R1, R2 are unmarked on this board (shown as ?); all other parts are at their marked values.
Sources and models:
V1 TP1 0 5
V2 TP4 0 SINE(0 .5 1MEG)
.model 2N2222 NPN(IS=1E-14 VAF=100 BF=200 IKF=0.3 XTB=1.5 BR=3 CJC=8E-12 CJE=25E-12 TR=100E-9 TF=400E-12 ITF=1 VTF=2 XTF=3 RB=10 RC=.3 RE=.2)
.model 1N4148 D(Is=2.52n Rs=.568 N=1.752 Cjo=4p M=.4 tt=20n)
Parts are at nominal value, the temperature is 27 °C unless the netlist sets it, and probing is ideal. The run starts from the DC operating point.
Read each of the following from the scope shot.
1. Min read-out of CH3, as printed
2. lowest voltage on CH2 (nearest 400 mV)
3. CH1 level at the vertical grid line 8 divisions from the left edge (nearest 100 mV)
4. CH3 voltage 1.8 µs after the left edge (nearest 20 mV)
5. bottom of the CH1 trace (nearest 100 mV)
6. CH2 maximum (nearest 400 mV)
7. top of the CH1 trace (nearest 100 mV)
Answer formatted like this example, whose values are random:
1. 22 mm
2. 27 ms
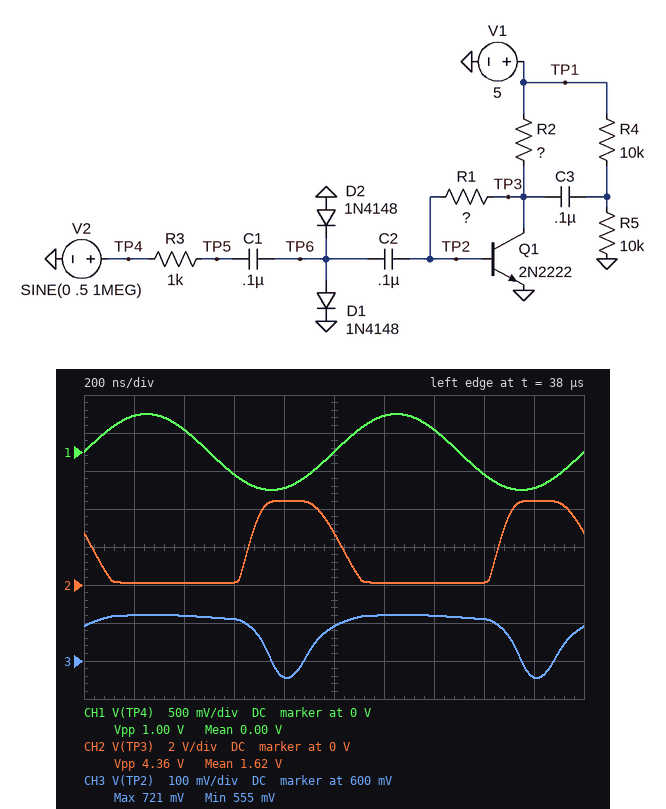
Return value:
1. 555 mV
2. 0 V
3. -300 mV
4. 560 mV
5. -500 mV
6. 4.4 V
7. 500 mV
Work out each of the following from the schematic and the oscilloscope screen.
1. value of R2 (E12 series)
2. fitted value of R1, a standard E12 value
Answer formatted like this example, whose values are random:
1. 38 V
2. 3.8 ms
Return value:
1. 560 Ω
2. 12 kΩ
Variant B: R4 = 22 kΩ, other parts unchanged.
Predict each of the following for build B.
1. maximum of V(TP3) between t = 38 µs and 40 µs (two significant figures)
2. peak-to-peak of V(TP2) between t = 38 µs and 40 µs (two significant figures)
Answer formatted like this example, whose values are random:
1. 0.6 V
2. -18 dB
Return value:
1. 4.5 V
2. 160 mV
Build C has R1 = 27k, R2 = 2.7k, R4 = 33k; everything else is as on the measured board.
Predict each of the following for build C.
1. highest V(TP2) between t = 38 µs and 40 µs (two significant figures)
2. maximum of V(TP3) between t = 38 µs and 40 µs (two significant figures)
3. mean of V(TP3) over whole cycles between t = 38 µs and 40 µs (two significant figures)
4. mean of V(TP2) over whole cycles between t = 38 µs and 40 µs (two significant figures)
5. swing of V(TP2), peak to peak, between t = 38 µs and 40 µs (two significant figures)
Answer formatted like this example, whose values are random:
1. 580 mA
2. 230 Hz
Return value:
1. 690 mV
2. 3.7 V
3. 1.5 V
4. 590 mV
5. 380 mV
